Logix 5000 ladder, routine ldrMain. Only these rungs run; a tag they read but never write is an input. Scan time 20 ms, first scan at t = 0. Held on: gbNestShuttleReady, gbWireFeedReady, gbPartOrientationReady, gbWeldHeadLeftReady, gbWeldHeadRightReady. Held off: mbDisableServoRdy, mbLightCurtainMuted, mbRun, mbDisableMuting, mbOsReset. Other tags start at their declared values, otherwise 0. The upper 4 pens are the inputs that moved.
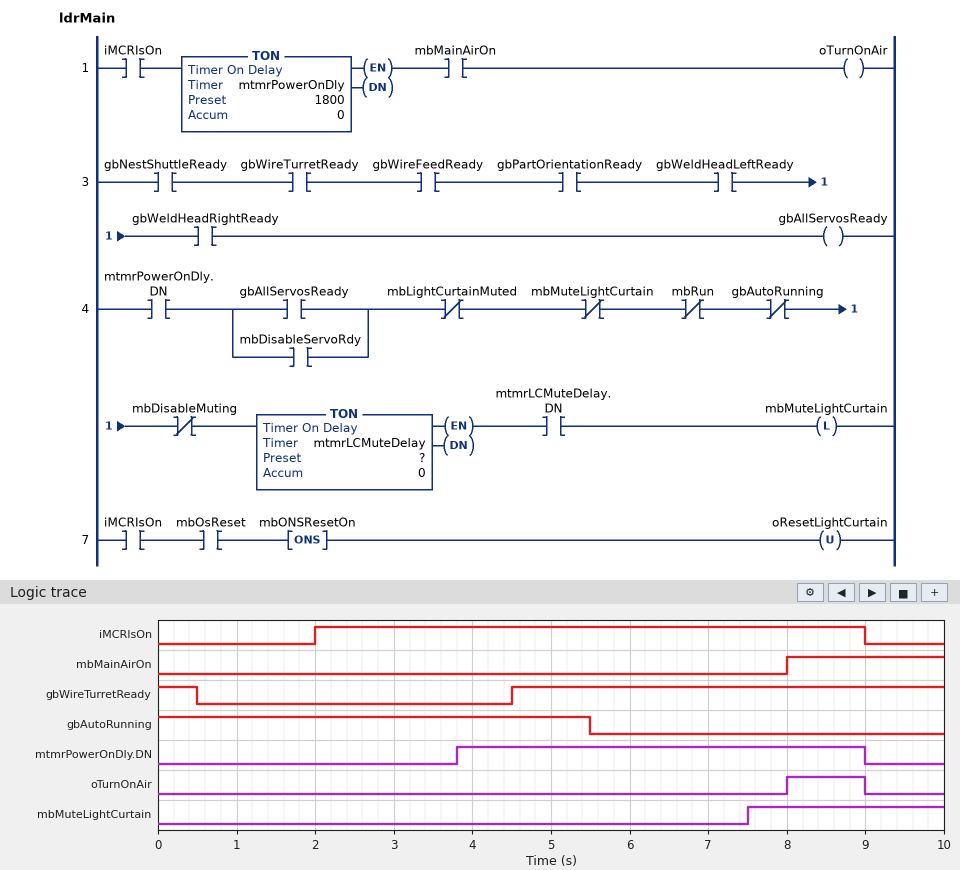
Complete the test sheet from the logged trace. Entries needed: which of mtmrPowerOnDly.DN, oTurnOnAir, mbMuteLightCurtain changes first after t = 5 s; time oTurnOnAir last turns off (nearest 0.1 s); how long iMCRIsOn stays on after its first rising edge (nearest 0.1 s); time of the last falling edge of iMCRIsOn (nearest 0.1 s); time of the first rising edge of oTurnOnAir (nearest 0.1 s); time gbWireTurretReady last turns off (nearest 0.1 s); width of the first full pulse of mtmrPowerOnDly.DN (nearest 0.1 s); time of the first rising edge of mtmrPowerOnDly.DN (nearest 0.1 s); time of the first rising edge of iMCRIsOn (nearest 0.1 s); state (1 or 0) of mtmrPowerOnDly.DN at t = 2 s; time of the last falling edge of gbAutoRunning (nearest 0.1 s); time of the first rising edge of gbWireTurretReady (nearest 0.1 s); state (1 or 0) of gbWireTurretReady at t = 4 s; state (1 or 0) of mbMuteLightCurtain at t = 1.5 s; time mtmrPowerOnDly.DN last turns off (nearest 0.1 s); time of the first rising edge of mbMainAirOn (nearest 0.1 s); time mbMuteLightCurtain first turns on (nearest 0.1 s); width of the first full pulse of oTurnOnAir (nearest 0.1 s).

mbMuteLightCurtain
9.0 s
7.0 s
9.0 s
8.0 s
0.5 s
5.2 s
3.8 s
2.0 s
0
5.5 s
4.5 s
0
0
9.0 s
8.0 s
7.5 s
1.0 s
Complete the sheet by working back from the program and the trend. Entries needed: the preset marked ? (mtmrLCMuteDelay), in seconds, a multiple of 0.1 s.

2.0 s
